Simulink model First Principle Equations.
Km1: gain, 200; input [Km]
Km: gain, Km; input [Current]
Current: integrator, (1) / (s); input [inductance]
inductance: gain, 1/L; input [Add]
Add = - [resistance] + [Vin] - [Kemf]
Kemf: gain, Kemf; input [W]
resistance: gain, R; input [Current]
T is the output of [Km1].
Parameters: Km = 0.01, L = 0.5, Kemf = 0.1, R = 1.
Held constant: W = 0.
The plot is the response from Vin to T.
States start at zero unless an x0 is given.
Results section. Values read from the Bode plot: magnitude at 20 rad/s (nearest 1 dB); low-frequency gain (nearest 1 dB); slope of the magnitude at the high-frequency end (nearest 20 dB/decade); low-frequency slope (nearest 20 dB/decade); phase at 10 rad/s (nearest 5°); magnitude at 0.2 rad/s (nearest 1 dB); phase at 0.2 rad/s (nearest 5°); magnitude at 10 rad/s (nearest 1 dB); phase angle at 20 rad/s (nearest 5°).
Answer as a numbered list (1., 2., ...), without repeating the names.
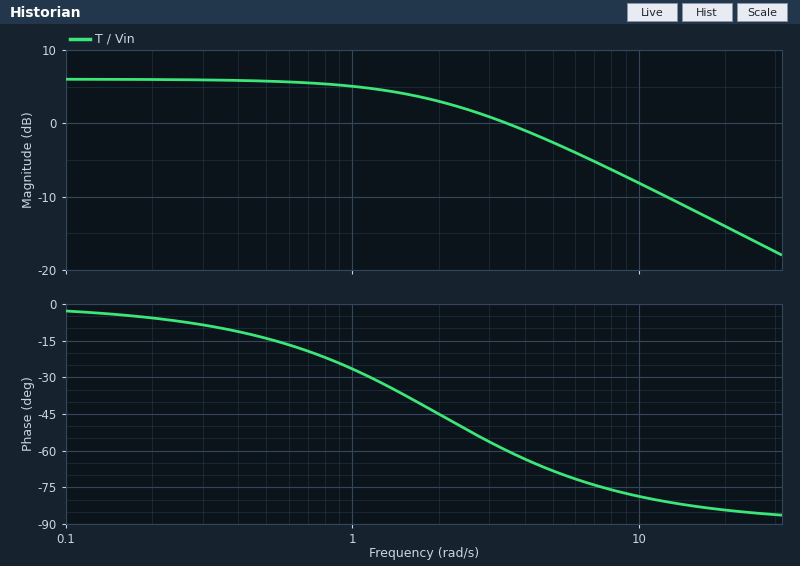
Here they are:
1. -14 dB
2. 6 dB
3. -20 dB/decade
4. 0 dB/decade
5. -80°
6. 6 dB
7. -5°
8. -8 dB
9. -85°
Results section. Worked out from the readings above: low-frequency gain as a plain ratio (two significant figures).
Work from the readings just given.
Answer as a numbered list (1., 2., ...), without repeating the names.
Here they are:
1. 2.0
